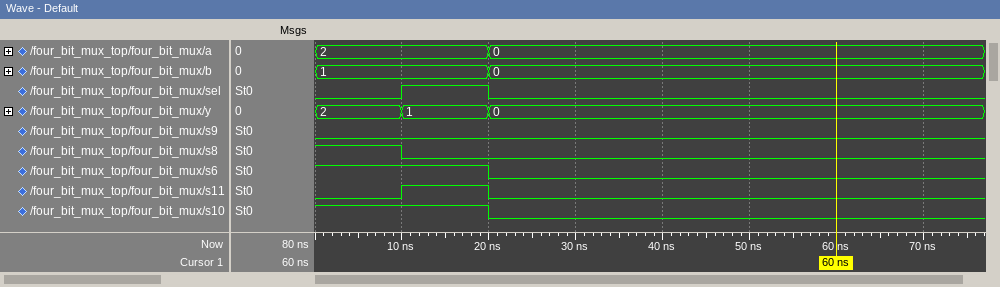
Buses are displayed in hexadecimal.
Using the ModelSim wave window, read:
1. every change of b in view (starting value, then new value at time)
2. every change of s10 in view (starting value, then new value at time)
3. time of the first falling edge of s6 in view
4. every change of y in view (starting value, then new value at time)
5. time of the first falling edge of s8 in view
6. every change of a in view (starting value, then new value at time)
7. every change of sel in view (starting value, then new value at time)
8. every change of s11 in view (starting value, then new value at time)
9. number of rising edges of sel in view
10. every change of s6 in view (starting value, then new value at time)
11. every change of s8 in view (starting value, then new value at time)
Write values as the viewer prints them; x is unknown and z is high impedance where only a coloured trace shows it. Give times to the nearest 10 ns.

1, 0 at 20 ns
1, 0 at 20 ns
20 ns
2, 1 at 10 ns, 0 at 20 ns
10 ns
2, 0 at 20 ns
0, 1 at 10 ns, 0 at 20 ns
0, 1 at 10 ns, 0 at 20 ns
1
1, 0 at 20 ns
1, 0 at 10 ns
